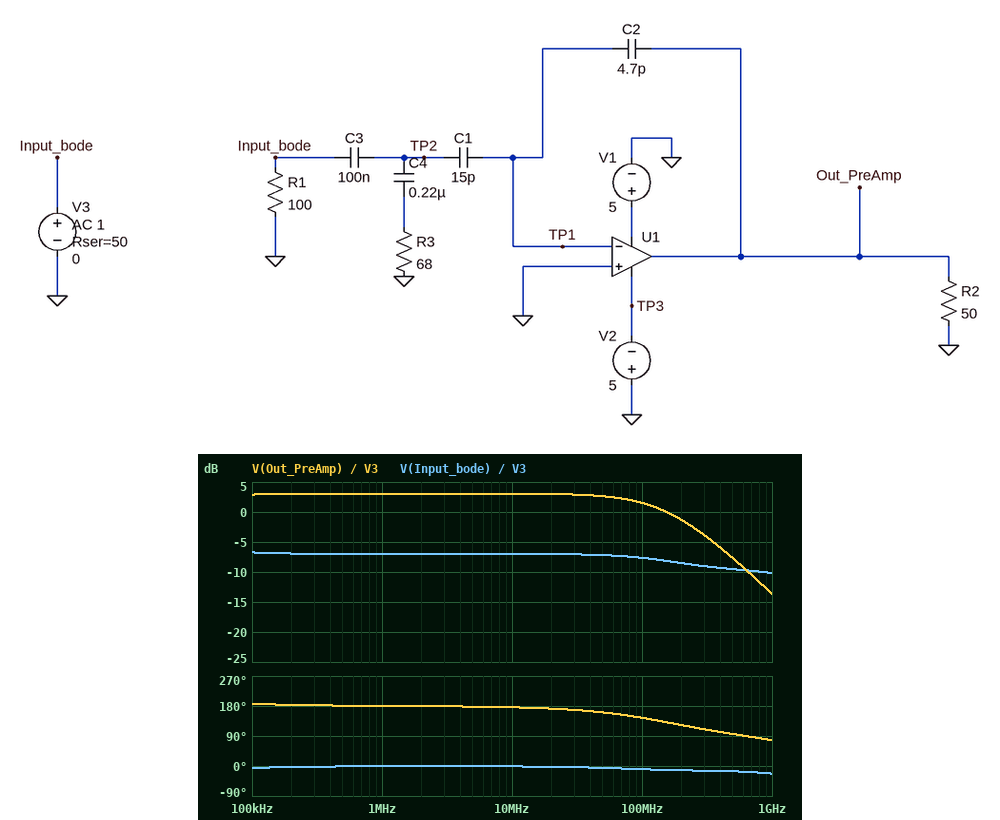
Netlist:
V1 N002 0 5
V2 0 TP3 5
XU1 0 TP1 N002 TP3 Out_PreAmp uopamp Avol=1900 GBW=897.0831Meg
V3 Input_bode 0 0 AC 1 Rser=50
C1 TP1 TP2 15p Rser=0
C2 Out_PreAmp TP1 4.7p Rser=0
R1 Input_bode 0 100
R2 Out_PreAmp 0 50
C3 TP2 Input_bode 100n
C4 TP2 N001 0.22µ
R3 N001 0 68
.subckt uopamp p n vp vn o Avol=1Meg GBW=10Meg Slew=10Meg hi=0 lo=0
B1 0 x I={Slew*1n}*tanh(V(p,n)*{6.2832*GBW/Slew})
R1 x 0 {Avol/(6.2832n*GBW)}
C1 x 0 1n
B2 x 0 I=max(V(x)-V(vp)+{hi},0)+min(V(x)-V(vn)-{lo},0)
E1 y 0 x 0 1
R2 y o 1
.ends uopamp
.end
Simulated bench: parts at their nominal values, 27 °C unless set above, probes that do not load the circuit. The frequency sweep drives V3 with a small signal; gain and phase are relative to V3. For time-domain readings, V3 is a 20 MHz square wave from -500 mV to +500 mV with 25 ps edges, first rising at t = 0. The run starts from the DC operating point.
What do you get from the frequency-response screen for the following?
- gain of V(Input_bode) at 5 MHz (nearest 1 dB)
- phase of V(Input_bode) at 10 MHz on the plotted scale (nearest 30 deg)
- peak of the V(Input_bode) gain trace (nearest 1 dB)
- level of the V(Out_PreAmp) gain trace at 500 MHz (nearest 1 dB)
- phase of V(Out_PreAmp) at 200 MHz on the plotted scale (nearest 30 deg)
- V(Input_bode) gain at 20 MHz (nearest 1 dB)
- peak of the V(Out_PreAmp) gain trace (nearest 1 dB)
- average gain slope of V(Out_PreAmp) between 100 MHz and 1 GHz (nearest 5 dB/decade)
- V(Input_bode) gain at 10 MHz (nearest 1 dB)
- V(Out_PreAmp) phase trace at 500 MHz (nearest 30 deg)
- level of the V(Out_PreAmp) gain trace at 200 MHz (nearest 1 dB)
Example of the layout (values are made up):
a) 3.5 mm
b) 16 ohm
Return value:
a) -7 dB
b) 0 deg
c) -7 dB
d) -8 dB
e) 120 deg
f) -7 dB
g) 3 dB
h) -15 dB/decade
i) -7 dB
j) 90 deg
k) -1 dB
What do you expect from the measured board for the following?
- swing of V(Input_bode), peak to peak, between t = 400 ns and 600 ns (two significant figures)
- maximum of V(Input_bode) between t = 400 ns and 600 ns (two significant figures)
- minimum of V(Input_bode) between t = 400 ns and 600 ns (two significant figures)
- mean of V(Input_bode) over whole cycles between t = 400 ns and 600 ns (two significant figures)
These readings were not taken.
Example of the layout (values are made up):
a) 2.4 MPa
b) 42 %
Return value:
a) 450 mV
b) 120 mV
c) -330 mV
d) -100 mV
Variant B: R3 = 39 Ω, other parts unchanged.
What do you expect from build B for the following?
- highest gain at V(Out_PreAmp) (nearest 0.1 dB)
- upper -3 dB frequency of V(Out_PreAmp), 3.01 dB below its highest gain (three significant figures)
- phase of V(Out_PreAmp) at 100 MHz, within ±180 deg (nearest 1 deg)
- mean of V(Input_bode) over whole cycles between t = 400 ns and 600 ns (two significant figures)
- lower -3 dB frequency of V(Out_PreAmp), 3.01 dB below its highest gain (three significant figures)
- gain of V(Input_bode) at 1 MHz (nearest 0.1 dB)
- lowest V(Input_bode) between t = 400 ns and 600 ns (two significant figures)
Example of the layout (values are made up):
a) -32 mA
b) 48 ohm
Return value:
a) 1.2 dB
b) 163 MHz
c) 147 deg
d) -140 mV
e) 18.3 kHz
f) -8.9 dB
g) -320 mV
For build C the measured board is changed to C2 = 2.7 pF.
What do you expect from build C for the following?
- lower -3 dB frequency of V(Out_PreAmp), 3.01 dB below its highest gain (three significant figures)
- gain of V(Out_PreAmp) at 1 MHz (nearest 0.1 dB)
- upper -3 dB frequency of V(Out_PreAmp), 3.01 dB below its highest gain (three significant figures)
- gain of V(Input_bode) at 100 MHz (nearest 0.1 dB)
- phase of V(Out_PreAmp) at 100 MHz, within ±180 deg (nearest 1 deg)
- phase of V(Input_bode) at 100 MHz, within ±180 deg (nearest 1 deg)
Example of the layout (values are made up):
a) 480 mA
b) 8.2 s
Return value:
a) 17.2 kHz
b) 7.9 dB
c) 108 MHz
d) -7.8 dB
e) 136 deg
f) -8 deg
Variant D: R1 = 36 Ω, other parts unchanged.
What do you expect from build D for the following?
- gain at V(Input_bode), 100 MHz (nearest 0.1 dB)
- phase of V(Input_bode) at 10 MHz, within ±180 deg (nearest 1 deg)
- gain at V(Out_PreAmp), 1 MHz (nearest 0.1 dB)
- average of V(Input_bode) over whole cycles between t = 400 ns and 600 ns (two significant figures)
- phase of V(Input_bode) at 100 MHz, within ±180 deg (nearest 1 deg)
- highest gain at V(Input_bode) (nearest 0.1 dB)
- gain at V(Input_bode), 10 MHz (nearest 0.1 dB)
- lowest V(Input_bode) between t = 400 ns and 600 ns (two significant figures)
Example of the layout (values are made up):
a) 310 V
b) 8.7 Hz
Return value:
a) -10.3 dB
b) -1 deg
c) 0.2 dB
d) -45 mV
e) -7 deg
f) -7.6 dB
g) -9.9 dB
h) -210 mV
